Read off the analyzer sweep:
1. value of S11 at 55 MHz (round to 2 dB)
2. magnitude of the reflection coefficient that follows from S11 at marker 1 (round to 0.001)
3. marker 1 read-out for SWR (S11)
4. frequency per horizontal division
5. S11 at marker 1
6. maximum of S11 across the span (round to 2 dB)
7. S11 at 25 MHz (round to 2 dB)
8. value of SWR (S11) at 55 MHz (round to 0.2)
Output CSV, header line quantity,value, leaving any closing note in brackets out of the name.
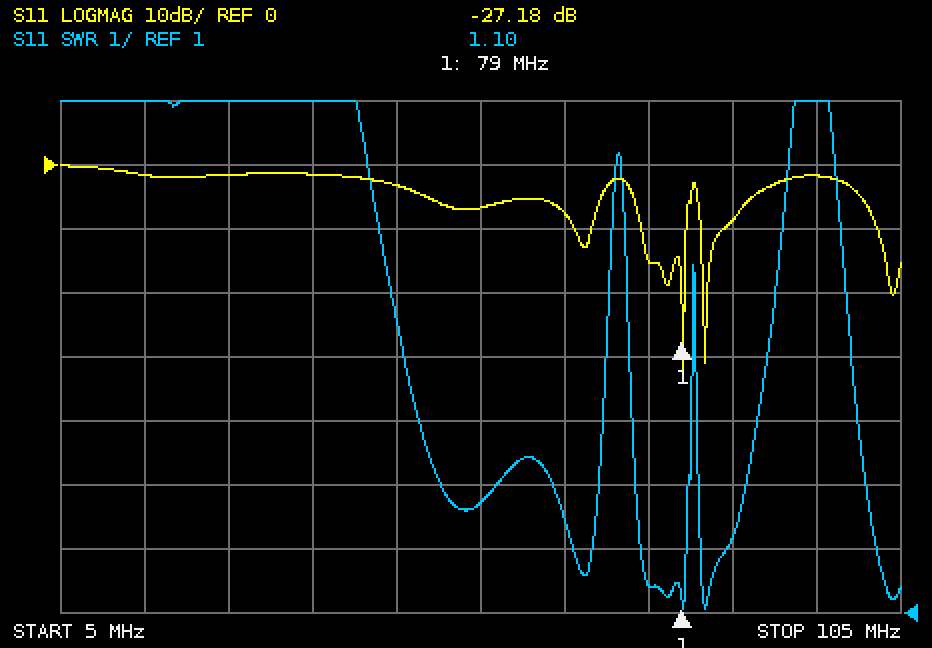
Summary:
quantity,value
value of S11 at 55 MHz,-6 dB
magnitude of the reflection coefficient that follows from S11 at marker 1,0.044
marker 1 read-out for SWR,1.10
frequency per horizontal division,10 MHz
S11 at marker 1,-27.18 dB
maximum of S11 across the span,0 dB
S11 at 25 MHz,-2 dB
value of SWR (S11) at 55 MHz,2.8
